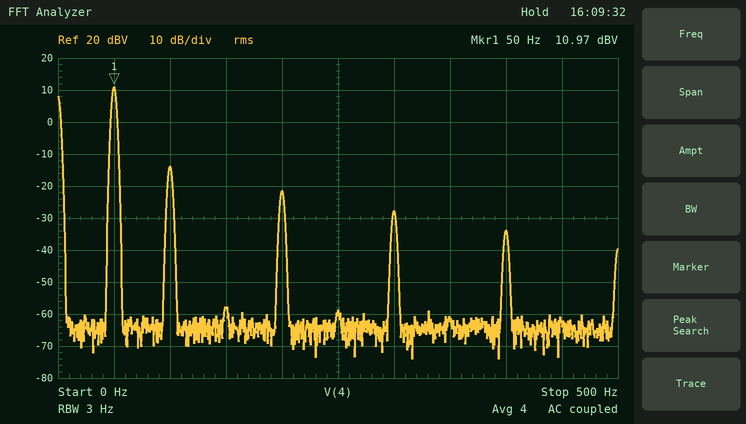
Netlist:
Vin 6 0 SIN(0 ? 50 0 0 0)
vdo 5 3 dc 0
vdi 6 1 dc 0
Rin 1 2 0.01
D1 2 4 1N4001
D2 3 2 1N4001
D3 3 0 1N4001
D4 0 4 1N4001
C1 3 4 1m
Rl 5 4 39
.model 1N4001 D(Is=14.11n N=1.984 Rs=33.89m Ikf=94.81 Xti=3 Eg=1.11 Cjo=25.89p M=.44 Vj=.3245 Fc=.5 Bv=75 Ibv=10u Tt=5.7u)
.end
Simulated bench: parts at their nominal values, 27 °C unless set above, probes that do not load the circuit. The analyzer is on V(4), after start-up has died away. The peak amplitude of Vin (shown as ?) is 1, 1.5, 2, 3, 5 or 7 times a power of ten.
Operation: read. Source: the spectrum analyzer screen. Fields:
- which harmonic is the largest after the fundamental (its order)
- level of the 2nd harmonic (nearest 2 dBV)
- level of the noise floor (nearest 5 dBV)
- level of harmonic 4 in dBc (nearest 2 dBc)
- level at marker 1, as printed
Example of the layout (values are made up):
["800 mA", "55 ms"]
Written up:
["2", "-14 dBV", "-65 dBV", "-32 dBc", "10.97 dBV"]
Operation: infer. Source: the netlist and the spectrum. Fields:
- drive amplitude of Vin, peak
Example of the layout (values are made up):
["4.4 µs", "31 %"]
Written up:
["10 V"]
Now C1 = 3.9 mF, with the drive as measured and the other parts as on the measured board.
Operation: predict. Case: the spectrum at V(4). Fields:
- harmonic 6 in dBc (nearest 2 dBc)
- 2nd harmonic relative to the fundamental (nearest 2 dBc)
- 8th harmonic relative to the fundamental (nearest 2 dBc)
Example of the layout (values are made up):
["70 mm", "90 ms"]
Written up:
["-48 dBc", "-36 dBc", "-52 dBc"]
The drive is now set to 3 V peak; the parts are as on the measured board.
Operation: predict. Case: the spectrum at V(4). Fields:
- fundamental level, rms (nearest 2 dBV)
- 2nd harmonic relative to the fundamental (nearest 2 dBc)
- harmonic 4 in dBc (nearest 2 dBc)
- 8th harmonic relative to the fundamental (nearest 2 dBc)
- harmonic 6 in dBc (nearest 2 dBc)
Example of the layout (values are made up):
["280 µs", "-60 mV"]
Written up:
["0 dBV", "-30 dBc", "-38 dBc", "-52 dBc", "-46 dBc"]
